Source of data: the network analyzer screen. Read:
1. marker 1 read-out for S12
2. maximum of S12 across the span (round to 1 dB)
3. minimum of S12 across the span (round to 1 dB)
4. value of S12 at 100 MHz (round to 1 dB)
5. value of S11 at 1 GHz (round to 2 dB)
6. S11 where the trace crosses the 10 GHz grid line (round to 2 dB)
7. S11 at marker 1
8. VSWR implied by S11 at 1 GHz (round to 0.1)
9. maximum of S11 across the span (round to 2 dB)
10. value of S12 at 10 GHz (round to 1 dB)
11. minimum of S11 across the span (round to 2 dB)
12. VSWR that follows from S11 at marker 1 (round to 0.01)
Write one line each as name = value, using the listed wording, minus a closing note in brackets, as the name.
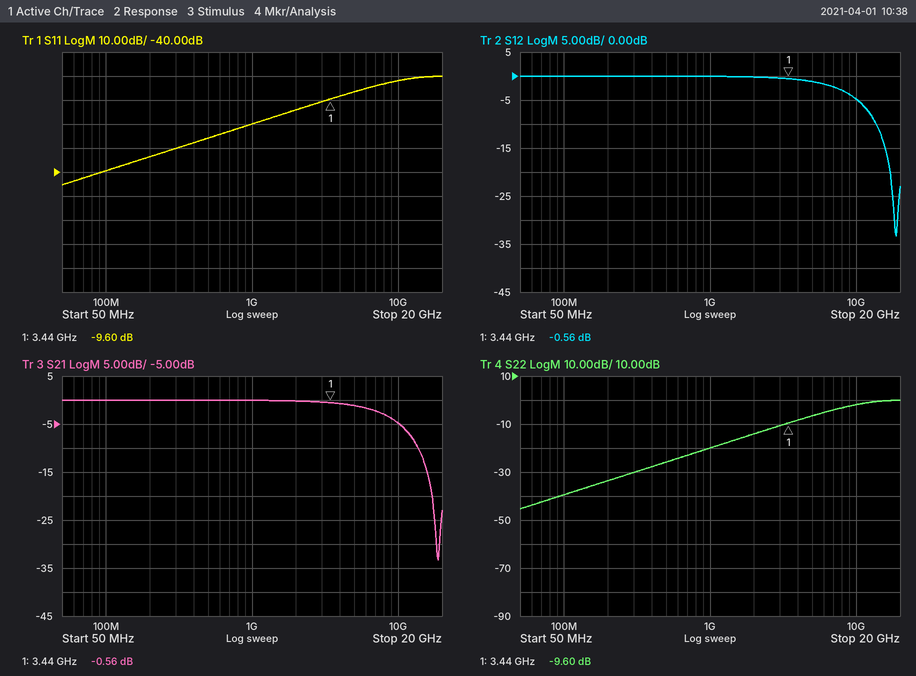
marker 1 read-out for S12 = -0.56 dB
maximum of S12 across the span = 0 dB
minimum of S12 across the span = -33 dB
value of S12 at 100 MHz = 0 dB
value of S11 at 1 GHz = -20 dB
S11 where the trace crosses the 10 GHz grid line = -2 dB
S11 at marker 1 = -9.60 dB
VSWR implied by S11 at 1 GHz = 1.2
maximum of S11 across the span = 0 dB
value of S12 at 10 GHz = -5 dB
minimum of S11 across the span = -46 dB
VSWR that follows from S11 at marker 1 = 1.99
